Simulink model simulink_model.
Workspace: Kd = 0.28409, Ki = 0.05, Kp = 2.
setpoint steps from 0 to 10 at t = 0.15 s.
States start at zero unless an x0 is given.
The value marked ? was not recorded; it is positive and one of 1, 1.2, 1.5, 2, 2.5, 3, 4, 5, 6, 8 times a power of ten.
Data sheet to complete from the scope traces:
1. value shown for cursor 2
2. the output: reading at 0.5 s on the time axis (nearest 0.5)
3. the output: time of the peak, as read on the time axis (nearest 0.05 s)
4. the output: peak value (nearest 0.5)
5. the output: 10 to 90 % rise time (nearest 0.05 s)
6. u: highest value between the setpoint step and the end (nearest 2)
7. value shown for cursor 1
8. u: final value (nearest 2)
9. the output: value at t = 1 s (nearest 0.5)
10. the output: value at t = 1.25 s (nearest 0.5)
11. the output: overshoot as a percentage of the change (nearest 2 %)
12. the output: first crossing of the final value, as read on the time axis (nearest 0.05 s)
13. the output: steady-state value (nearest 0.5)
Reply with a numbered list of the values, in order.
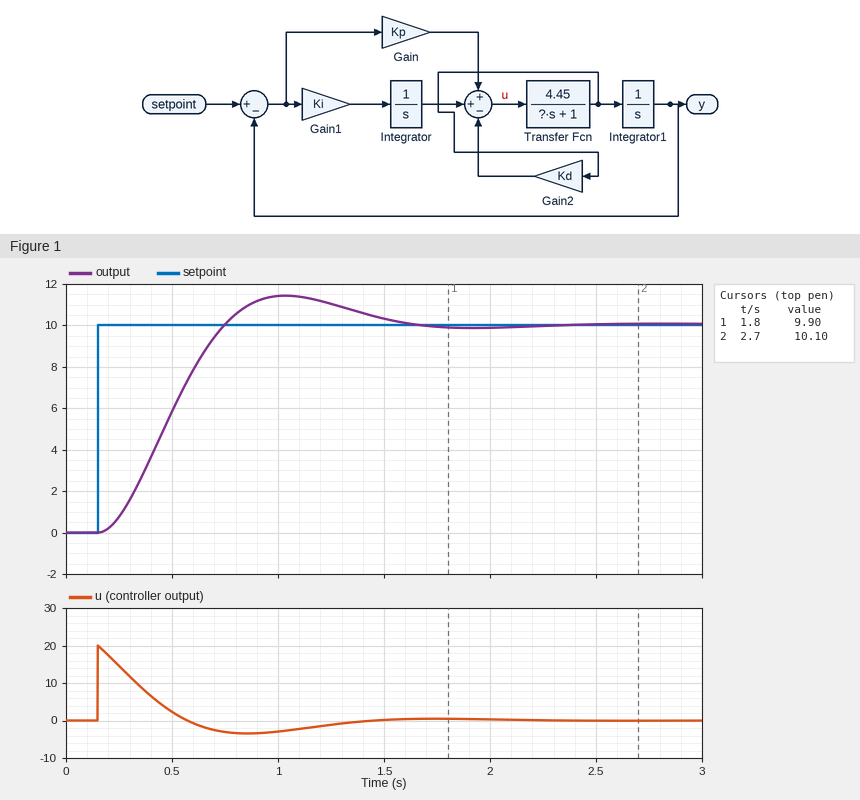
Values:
1. 10.10
2. 6.0
3. 1.05 s
4. 11.5
5. 0.40 s
6. 20
7. 9.90
8. 0
9. 11.5
10. 11.0
11. 14 %
12. 0.75 s
13. 10.0
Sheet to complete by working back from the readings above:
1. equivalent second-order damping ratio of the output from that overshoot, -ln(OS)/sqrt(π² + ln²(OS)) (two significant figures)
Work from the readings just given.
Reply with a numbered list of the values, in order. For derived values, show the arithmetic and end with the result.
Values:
1. ln(0.14) = -1.966; 1.966 / sqrt(9.870 + 3.866) = 0.53
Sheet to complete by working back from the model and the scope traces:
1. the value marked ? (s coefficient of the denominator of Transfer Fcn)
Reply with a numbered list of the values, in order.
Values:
1. 0.5
